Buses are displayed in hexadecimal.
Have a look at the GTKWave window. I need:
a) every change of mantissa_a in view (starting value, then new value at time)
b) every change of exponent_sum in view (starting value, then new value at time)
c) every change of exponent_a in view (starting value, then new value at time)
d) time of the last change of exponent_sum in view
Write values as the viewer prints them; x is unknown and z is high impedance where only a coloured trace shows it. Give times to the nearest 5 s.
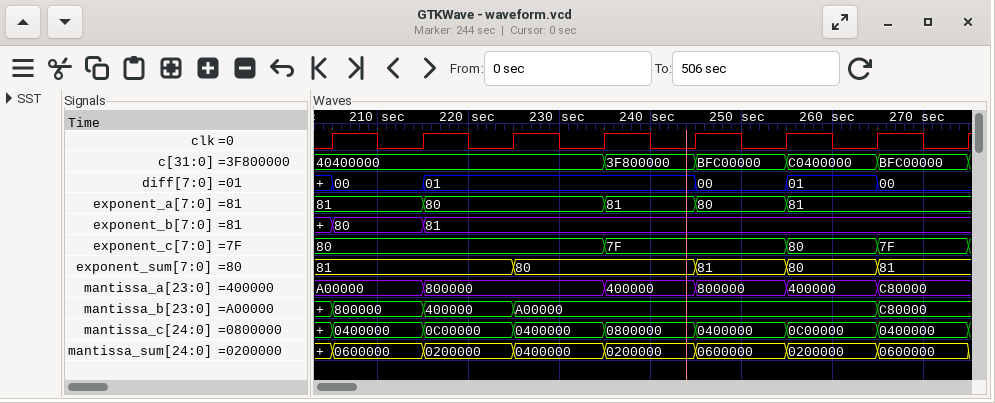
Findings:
A00000, 800000 at 215 s, 400000 at 235 s, 800000 at 245 s, 400000 at 255 s, C80000 at 265 s
81, 80 at 225 s, 81 at 245 s, 80 at 255 s, 81 at 265 s
81, 80 at 215 s, 81 at 235 s, 80 at 245 s, 81 at 255 s
265 s
